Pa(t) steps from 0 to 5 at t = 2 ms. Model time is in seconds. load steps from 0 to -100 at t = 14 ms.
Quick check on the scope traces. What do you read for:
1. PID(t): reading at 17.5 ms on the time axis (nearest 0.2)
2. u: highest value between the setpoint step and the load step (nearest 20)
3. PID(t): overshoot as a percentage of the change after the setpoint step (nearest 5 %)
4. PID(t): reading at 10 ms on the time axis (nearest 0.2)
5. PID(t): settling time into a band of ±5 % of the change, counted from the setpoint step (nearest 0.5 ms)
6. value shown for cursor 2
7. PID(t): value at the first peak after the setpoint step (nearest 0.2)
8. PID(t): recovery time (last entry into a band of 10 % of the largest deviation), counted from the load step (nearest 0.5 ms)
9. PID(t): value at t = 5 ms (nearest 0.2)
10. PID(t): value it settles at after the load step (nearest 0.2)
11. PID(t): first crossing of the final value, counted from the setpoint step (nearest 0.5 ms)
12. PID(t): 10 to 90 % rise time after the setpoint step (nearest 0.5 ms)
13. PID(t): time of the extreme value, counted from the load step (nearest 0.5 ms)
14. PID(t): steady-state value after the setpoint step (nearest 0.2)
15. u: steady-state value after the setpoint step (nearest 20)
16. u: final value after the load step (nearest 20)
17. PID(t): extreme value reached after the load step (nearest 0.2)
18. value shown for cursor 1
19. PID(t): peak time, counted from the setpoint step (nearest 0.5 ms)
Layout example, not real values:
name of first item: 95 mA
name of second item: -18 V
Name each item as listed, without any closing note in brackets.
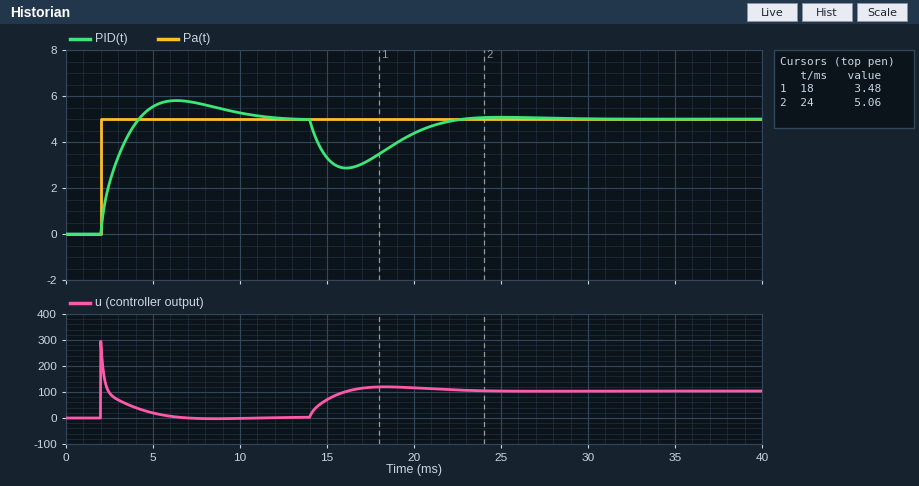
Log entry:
PID(t): reading at 17.5 ms on the time axis: 3.2
u: highest value between the setpoint step and the load step: 300
PID(t): overshoot as a percentage of the change after the setpoint step: 15 %
PID(t): reading at 10 ms on the time axis: 5.2
PID(t): settling time into a band of ±5 % of the change, counted from the setpoint step: 8.0 ms
value shown for cursor 2: 5.06
PID(t): value at the first peak after the setpoint step: 5.8
PID(t): recovery time (last entry into a band of 10 % of the largest deviation), counted from the load step: 7.5 ms
PID(t): value at t = 5 ms: 5.6
PID(t): value it settles at after the load step: 5.0
PID(t): first crossing of the final value, counted from the setpoint step: 2.0 ms
PID(t): 10 to 90 % rise time after the setpoint step: 1.5 ms
PID(t): time of the extreme value, counted from the load step: 2.0 ms
PID(t): steady-state value after the setpoint step: 5.0
u: steady-state value after the setpoint step: 0
u: final value after the load step: 100
PID(t): extreme value reached after the load step: 2.8
value shown for cursor 1: 3.48
PID(t): peak time, counted from the setpoint step: 4.5 ms
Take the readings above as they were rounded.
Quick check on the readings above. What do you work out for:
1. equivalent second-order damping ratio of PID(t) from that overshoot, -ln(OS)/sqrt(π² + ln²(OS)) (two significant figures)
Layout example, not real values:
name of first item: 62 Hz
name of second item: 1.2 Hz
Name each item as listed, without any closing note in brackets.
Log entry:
equivalent second-order damping ratio of PID(t) from that overshoot, -ln(OS)/sqrt(π² + ln²(OS)): 0.52
